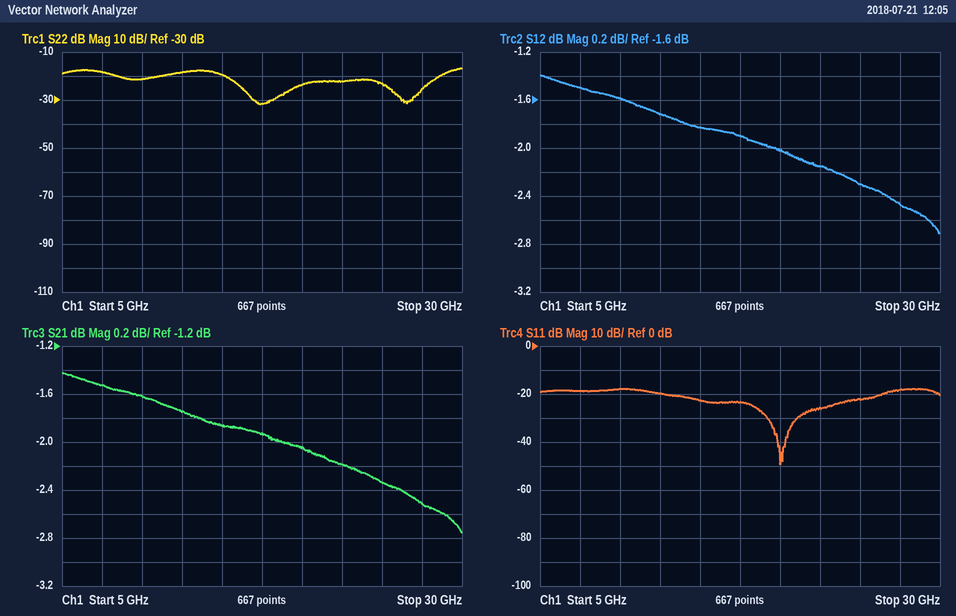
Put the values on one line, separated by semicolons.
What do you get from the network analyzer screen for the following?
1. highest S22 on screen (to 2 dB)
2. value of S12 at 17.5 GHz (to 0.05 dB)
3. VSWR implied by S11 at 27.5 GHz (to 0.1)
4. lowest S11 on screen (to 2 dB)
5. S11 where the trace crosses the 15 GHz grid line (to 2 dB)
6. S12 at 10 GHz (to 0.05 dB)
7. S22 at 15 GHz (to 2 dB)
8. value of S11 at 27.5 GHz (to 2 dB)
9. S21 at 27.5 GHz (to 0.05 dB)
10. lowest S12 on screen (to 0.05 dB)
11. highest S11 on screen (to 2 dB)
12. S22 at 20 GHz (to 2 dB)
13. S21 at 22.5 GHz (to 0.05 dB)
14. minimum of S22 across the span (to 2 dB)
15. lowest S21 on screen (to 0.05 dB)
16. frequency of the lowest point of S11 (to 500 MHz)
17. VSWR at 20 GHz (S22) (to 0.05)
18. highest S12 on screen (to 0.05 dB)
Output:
-16 dB; -1.90 dB; 1.3; -50 dB; -22 dB; -1.60 dB; -20 dB; -18 dB; -2.50 dB; -2.70 dB; -18 dB; -24 dB; -2.20 dB; -32 dB; -2.75 dB; 20.0 GHz; 1.15; -1.40 dB
